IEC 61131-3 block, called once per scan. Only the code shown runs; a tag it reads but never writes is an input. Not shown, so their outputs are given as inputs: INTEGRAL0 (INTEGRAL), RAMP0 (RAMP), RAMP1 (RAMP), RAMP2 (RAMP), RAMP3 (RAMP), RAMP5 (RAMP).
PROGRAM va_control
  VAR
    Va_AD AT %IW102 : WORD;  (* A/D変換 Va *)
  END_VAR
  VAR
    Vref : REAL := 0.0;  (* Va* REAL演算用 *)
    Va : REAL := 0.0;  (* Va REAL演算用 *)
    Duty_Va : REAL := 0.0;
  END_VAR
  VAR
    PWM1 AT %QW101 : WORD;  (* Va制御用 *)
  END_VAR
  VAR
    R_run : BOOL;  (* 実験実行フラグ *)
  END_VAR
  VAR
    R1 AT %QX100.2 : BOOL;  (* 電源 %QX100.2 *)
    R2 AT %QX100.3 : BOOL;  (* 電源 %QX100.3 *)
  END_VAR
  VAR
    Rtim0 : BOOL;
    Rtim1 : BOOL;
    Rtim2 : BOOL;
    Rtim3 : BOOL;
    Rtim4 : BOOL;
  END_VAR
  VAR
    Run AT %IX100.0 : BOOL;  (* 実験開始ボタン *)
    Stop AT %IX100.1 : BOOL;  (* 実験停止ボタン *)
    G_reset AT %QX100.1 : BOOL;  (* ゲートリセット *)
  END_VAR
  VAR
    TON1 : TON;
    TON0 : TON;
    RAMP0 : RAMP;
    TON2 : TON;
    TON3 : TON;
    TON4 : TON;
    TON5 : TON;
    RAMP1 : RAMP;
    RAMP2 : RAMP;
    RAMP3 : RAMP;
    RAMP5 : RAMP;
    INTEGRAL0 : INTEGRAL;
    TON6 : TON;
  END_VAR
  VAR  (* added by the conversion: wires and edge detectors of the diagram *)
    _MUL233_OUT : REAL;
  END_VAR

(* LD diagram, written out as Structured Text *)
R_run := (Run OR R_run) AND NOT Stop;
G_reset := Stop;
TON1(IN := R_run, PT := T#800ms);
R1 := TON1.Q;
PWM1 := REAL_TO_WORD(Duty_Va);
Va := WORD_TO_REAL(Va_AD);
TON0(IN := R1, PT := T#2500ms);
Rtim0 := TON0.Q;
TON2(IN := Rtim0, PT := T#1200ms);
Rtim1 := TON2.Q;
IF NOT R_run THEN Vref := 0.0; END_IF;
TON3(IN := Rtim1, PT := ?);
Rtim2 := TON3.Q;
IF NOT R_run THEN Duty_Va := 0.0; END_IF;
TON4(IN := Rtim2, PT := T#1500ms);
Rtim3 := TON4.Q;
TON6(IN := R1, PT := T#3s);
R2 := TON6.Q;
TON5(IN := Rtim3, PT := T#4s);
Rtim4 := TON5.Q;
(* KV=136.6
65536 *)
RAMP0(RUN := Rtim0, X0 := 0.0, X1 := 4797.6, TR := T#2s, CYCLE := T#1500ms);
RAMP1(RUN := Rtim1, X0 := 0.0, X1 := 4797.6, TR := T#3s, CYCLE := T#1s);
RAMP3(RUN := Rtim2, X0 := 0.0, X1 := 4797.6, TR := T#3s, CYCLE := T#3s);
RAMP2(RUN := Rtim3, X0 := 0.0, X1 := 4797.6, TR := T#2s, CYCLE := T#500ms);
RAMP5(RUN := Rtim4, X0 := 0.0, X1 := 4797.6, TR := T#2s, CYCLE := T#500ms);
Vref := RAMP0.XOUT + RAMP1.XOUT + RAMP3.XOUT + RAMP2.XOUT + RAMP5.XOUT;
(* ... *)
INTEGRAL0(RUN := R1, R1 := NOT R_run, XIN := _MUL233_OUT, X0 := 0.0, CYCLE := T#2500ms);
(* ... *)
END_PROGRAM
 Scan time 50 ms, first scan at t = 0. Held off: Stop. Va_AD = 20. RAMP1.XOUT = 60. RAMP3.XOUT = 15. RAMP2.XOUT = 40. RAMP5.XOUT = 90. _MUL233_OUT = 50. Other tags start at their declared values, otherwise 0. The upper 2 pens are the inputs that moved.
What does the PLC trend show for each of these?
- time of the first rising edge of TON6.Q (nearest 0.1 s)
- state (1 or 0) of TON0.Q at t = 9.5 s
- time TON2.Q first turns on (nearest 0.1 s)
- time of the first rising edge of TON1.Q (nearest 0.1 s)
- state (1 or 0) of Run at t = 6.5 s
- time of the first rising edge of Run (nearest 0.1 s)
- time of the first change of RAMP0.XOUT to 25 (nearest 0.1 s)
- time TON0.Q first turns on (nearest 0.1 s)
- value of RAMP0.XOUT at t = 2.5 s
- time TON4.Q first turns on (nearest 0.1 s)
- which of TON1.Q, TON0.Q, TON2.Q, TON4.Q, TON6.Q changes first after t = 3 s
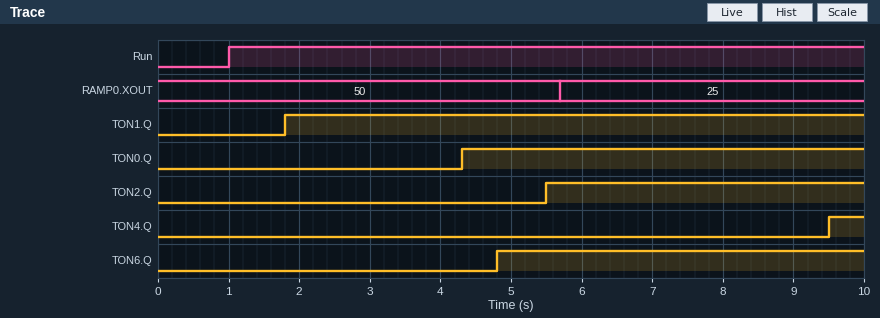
4.8 s
1
5.5 s
1.8 s
1
1.0 s
5.7 s
4.3 s
50
9.5 s
TON0.Q
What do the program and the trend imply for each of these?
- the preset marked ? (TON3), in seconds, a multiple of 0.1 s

2.5 s
